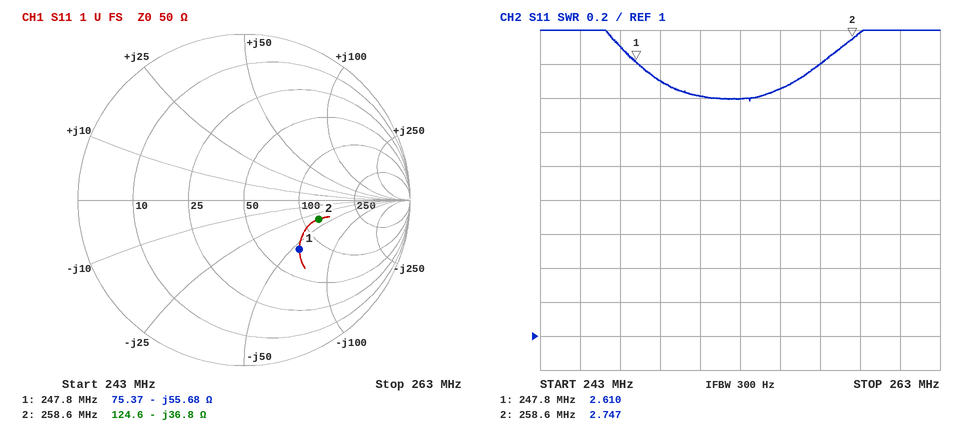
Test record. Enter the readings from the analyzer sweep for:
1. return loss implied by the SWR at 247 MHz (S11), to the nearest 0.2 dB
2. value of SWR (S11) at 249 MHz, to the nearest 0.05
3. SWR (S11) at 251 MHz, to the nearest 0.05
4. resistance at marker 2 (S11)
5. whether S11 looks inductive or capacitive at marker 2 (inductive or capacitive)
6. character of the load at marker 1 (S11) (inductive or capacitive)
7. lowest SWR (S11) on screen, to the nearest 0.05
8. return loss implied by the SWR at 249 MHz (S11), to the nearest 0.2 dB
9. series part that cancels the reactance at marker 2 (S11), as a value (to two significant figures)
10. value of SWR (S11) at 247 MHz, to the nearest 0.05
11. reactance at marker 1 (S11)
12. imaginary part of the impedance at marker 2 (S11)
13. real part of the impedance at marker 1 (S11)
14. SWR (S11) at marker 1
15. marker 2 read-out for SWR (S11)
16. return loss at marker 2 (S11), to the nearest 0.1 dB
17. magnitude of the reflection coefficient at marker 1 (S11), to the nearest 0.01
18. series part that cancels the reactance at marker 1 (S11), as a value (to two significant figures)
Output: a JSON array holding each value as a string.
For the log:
["6.8 dB", "2.50", "2.40", "124.6 Ω", "capacitive", "capacitive", "2.40", "7.4 dB", "23 nH", "2.70", "-55.68 Ω", "-36.8 Ω", "75.37 Ω", "2.610", "2.747", "6.6 dB", "0.45", "36 nH"]
